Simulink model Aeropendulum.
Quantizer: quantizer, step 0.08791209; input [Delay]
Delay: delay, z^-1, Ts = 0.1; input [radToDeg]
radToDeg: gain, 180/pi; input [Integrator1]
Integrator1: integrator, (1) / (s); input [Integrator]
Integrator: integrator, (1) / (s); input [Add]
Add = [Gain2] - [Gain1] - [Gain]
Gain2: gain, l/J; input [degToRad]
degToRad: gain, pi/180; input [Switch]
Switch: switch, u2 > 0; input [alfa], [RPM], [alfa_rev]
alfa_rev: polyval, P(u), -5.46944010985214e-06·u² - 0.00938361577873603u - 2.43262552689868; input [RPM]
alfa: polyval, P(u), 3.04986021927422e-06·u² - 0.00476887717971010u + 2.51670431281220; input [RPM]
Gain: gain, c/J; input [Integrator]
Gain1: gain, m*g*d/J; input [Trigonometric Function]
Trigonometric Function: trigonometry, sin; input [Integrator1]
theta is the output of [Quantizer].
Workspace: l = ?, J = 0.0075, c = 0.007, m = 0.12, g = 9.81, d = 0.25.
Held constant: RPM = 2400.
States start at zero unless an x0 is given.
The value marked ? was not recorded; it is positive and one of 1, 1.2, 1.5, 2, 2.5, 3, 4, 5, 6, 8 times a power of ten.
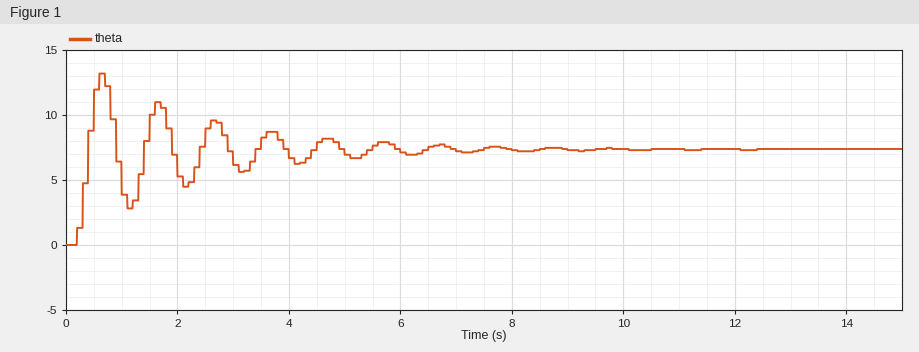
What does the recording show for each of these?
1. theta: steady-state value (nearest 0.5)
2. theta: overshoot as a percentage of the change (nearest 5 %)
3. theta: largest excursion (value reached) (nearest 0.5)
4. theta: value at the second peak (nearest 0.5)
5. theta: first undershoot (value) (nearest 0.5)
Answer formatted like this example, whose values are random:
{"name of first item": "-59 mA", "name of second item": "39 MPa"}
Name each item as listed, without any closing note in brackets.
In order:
{"theta: steady-state value": "7.5", "theta: overshoot as a percentage of the change": "80 %", "theta: largest excursion (value reached)": "13.0", "theta: value at the second peak": "11.0", "theta: first undershoot (value)": "3.0"}
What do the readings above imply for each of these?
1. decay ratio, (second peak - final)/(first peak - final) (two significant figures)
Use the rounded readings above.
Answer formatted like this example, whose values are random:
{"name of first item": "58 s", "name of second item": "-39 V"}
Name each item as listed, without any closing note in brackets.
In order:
{"decay ratio, (second peak - final)/(first peak - final)": "0.64"}
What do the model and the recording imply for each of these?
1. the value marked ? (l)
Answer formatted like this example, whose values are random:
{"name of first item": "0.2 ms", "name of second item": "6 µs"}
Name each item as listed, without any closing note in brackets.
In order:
{"the value marked ?": "0.25"}
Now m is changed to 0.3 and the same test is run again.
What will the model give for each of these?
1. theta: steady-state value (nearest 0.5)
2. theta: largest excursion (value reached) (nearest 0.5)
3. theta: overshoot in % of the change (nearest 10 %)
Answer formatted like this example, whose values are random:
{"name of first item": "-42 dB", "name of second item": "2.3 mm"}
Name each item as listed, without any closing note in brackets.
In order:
{"theta: steady-state value": "3.0", "theta: largest excursion (value reached)": "5.5", "theta: overshoot in % of the change": "90 %"}
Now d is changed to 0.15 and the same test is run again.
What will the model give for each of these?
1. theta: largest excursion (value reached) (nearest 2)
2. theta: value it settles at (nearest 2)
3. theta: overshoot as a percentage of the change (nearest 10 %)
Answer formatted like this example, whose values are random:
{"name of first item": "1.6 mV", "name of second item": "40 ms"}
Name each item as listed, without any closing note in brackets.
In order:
{"theta: largest excursion (value reached)": "22", "theta: value it settles at": "12", "theta: overshoot as a percentage of the change": "70 %"}
